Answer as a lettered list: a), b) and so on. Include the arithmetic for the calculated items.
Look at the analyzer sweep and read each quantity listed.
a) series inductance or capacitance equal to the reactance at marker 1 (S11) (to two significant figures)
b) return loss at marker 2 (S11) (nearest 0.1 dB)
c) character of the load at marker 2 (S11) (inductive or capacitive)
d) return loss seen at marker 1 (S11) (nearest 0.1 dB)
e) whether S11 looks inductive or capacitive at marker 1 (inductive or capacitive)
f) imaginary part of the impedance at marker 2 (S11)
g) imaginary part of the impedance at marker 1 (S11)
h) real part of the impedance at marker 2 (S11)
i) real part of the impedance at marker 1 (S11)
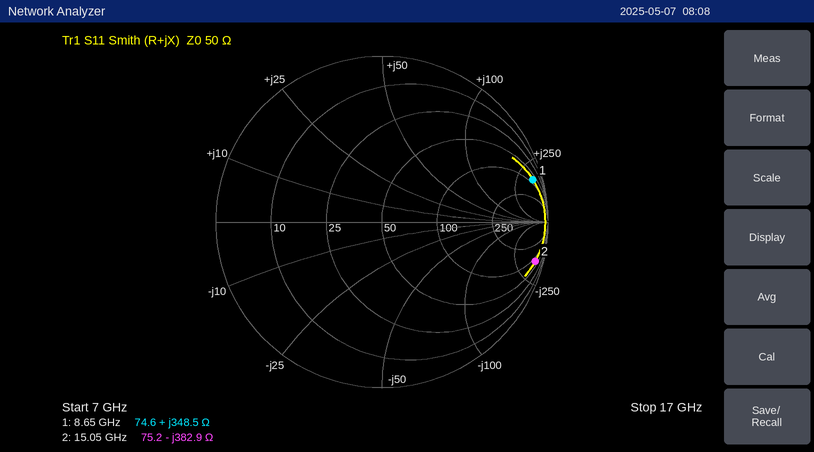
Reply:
a) L = 348.5 Ω/(2π × 8.65 GHz) ≈ 6.4 nH
b) 0.4 dB
c) capacitive
d) 0.5 dB
e) inductive
f) -382.9 Ω
g) +348.5 Ω
h) 75.2 Ω
i) 74.6 Ω
